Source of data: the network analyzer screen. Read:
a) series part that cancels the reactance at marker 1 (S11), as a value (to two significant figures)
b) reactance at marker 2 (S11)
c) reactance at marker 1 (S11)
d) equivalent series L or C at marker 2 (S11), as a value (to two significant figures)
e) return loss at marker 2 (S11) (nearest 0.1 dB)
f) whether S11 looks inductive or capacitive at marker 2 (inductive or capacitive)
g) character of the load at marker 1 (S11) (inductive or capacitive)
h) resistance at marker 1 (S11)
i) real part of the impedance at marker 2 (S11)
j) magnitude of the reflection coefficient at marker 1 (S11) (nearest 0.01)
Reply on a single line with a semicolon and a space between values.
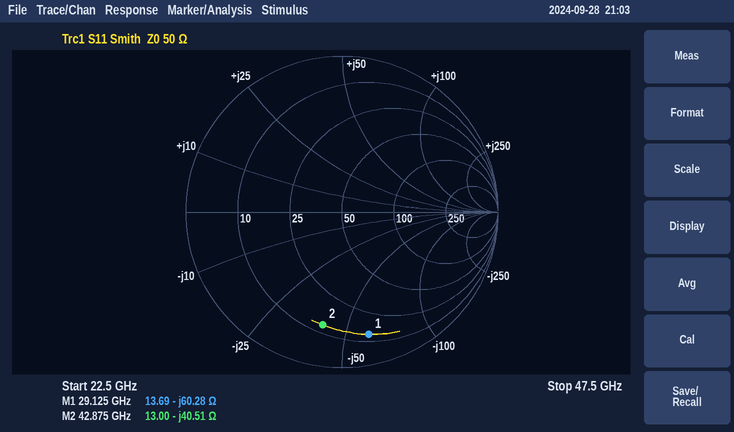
330 pH; -40.51 Ω; -60.28 Ω; 92 fF; 2.7 dB; capacitive; capacitive; 13.69 Ω; 13.00 Ω; 0.80
